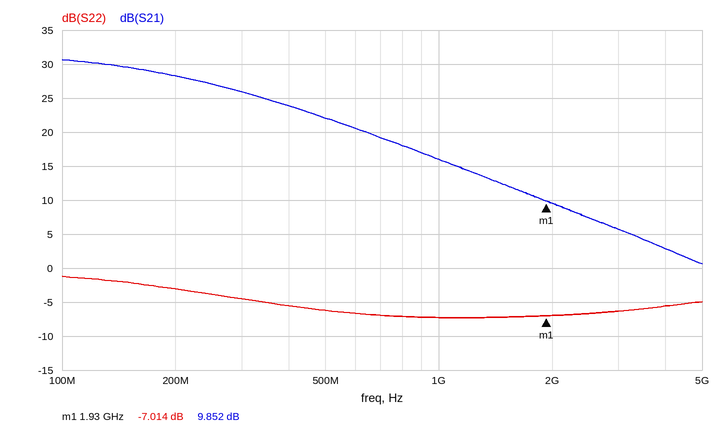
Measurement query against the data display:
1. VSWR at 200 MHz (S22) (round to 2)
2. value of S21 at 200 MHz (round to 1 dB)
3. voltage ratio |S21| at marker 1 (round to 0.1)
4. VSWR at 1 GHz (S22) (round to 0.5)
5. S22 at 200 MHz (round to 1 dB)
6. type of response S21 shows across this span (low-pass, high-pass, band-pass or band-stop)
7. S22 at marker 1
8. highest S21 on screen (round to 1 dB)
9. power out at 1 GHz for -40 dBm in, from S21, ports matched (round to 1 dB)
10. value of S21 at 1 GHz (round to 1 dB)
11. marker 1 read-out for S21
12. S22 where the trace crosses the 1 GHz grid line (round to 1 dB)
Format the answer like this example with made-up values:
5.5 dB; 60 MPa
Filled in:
6; 28 dB; 3.1; 2.5; -3 dB; low-pass; -7.014 dB; 31 dB; -24 dBm; 16 dB; 9.852 dB; -7 dB
